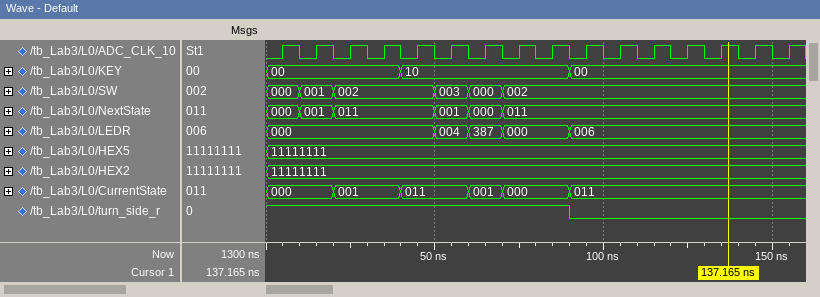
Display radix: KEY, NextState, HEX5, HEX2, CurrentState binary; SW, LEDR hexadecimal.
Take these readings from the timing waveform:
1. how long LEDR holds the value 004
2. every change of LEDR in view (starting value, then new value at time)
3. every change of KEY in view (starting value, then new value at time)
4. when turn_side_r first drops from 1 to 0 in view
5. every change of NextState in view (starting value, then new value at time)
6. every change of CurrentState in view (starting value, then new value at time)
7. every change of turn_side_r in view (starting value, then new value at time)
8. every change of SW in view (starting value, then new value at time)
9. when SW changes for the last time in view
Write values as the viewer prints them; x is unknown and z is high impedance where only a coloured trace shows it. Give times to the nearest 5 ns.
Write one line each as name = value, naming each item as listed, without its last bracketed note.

how long LEDR holds the value 004 = 10 ns
every change of LEDR in view = 000, 004 at 50 ns, 387 at 60 ns, 000 at 70 ns, 006 at 90 ns
every change of KEY in view = 00, 10 at 40 ns, 00 at 90 ns
when turn_side_r first drops from 1 to 0 in view = 90 ns
every change of NextState in view = 000, 001 at 10 ns, 011 at 20 ns, 001 at 50 ns, 000 at 60 ns, 011 at 70 ns
every change of CurrentState in view = 000, 001 at 20 ns, 011 at 40 ns, 001 at 60 ns, 000 at 70 ns, 011 at 90 ns
every change of turn_side_r in view = 1, 0 at 90 ns
every change of SW in view = 000, 001 at 10 ns, 002 at 20 ns, 003 at 50 ns, 000 at 60 ns, 002 at 70 ns
when SW changes for the last time in view = 70 ns
